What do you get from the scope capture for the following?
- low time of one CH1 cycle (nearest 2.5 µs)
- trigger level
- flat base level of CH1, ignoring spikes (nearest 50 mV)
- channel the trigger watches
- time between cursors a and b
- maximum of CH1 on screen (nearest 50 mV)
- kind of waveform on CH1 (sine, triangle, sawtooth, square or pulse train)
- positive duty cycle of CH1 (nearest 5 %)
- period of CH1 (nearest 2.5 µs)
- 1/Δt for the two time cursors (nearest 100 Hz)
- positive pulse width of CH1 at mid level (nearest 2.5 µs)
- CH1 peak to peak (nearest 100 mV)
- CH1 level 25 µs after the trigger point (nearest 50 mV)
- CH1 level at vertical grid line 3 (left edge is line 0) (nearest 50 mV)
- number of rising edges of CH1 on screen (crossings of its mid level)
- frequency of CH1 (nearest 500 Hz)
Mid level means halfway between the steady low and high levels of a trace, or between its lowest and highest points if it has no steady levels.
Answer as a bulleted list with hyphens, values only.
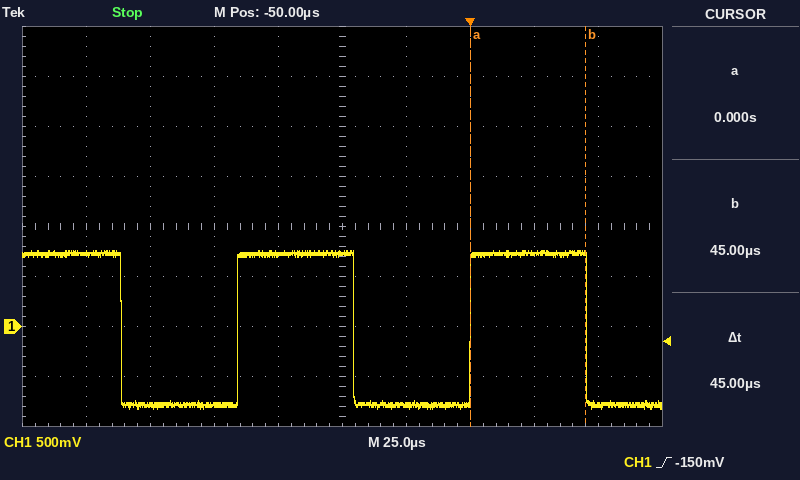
- 45.0 µs
- -150 mV
- -800 mV
- CH1
- 45 µs
- 750 mV
- square
- 50 %
- 90.0 µs
- 22.2 kHz
- 45.0 µs
- 1.60 V
- 750 mV
- -800 mV
- 2
- 11.0 kHz
